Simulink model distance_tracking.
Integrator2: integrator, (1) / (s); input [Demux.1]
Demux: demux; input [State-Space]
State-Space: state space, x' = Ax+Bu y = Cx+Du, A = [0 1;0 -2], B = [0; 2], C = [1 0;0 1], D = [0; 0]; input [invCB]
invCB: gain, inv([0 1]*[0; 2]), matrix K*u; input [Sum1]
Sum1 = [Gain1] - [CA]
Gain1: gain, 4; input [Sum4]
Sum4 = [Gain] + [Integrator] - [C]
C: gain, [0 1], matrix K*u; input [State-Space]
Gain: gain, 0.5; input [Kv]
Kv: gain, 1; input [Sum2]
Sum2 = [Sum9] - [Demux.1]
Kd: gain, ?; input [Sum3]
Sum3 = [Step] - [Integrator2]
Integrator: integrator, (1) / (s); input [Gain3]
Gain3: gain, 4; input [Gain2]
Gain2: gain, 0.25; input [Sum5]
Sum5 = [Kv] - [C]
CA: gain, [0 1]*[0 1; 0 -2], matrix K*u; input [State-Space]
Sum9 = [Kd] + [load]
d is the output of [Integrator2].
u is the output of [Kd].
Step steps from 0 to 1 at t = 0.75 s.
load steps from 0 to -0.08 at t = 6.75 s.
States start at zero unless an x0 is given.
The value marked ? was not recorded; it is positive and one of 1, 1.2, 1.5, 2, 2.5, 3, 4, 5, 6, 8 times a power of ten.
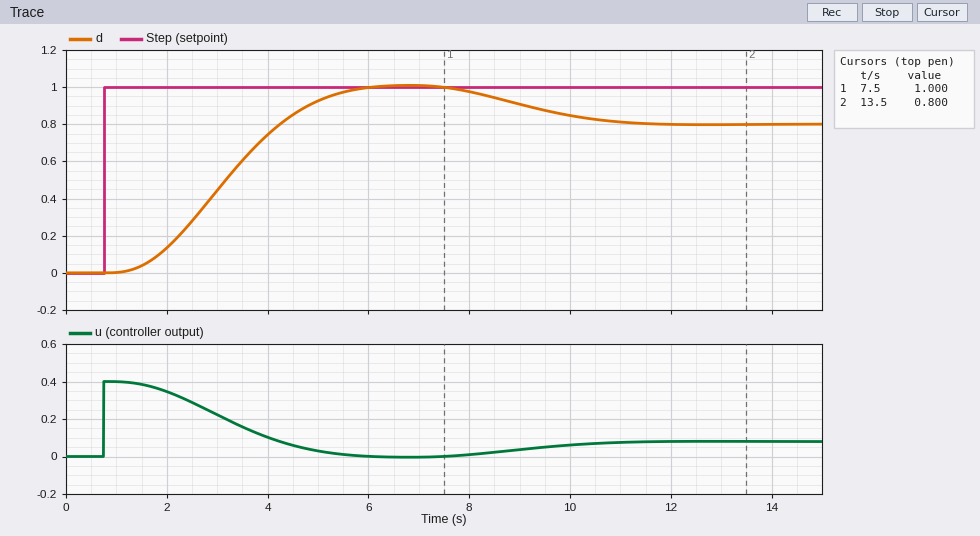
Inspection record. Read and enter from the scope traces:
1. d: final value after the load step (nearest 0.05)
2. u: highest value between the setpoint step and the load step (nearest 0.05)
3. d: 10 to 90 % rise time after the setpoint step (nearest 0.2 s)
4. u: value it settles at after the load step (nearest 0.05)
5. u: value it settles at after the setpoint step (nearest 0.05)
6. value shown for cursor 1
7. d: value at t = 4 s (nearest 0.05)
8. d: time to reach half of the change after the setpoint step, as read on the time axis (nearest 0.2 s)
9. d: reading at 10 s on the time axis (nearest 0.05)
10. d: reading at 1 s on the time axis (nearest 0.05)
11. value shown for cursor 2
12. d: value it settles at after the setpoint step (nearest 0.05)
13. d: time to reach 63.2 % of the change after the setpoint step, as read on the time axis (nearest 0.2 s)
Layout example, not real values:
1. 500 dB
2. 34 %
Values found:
1. 0.80
2. 0.40
3. 3.0 s
4. 0.10
5. 0.00
6. 1.000
7. 0.75
8. 3.2 s
9. 0.85
10. 0.00
11. 0.800
12. 1.00
13. 3.6 s
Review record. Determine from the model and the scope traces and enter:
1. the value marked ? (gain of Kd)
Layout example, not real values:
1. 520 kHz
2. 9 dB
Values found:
1. 0.4
